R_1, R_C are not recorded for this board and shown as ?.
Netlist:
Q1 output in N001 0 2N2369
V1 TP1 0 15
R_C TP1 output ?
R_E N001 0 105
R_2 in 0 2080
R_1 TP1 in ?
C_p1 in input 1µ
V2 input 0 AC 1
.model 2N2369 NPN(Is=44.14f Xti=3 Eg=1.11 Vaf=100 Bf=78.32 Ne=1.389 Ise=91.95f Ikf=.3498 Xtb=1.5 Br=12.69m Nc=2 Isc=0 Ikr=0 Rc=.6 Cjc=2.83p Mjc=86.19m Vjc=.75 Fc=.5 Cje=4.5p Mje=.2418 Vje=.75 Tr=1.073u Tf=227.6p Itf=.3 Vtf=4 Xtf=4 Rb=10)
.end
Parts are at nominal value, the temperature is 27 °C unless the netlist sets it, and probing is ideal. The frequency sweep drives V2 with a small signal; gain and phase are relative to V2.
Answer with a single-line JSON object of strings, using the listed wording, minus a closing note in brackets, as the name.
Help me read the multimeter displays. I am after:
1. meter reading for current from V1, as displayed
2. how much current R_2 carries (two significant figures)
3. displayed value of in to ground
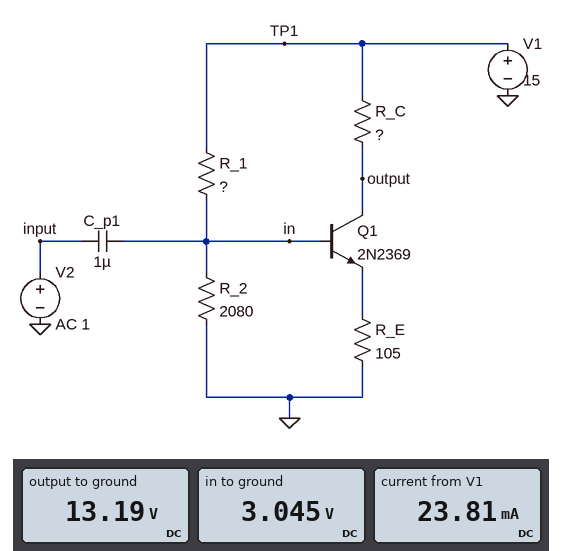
{"meter reading for current from V1, as displayed": "23.81 mA", "how much current R_2 carries": "1.5 mA", "displayed value of in to ground": "3.045 V"}
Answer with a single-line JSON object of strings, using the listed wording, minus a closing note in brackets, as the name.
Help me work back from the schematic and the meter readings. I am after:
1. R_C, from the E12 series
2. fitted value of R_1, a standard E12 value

{"R_C, from the E12 series": "82 Ω", "fitted value of R_1, a standard E12 value": "6.8 kΩ"}
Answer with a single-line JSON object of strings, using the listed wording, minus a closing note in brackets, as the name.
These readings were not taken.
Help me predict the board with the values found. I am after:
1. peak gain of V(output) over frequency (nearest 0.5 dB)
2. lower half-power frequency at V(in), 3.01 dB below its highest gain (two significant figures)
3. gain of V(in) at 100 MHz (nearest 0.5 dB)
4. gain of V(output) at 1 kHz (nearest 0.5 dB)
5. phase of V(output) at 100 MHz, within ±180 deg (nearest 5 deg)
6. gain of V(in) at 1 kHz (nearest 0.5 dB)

{"peak gain of V(output) over frequency": "-1.5 dB", "lower half-power frequency at V(in), 3.01 dB below its highest gain": "120 Hz", "gain of V(in) at 100 MHz": "0 dB", "gain of V(output) at 1 kHz": "-2.5 dB", "phase of V(output) at 100 MHz, within ±180 deg": "155 deg", "gain of V(in) at 1 kHz": "0 dB"}
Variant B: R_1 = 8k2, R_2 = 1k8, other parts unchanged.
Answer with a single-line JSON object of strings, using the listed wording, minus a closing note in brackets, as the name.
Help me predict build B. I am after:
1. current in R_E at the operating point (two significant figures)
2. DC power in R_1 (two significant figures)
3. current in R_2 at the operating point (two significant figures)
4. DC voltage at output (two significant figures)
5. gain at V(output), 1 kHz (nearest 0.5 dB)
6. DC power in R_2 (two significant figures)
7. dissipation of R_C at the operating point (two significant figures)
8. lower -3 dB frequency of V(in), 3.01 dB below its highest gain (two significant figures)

{"current in R_E at the operating point": "16 mA", "DC power in R_1": "19 mW", "current in R_2 at the operating point": "1.3 mA", "DC voltage at output": "14 V", "gain at V(output), 1 kHz": "-2.5 dB", "DC power in R_2": "3.2 mW", "dissipation of R_C at the operating point": "21 mW", "lower -3 dB frequency of V(in), 3.01 dB below its highest gain": "130 Hz"}
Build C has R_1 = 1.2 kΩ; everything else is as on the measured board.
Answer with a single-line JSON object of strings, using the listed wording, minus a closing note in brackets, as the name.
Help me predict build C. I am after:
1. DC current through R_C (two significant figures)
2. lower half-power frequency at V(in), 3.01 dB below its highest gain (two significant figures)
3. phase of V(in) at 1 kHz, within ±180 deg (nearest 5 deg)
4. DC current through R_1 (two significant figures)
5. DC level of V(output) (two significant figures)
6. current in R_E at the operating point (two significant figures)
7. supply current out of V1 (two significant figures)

{"DC current through R_C": "74 mA", "lower half-power frequency at V(in), 3.01 dB below its highest gain": "240 Hz", "phase of V(in) at 1 kHz, within ±180 deg": "15 deg", "DC current through R_1": "5.3 mA", "DC level of V(output)": "9.0 V", "current in R_E at the operating point": "75 mA", "supply current out of V1": "79 mA"}
